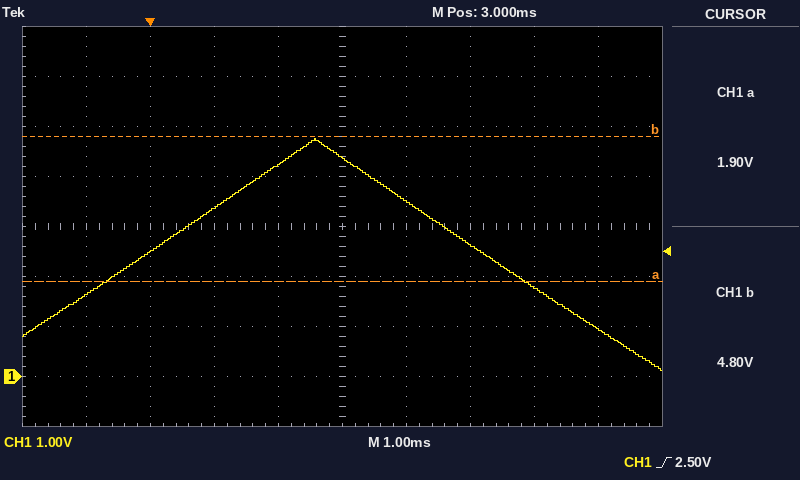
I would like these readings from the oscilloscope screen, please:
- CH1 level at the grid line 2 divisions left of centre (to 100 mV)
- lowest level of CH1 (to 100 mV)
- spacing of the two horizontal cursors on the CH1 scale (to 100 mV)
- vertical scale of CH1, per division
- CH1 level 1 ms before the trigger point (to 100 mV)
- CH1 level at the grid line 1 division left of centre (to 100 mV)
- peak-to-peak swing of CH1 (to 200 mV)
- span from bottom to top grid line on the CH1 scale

3.4 V
100 mV
2.9 V
1 V
1.6 V
4.2 V
4.6 V
8 V
